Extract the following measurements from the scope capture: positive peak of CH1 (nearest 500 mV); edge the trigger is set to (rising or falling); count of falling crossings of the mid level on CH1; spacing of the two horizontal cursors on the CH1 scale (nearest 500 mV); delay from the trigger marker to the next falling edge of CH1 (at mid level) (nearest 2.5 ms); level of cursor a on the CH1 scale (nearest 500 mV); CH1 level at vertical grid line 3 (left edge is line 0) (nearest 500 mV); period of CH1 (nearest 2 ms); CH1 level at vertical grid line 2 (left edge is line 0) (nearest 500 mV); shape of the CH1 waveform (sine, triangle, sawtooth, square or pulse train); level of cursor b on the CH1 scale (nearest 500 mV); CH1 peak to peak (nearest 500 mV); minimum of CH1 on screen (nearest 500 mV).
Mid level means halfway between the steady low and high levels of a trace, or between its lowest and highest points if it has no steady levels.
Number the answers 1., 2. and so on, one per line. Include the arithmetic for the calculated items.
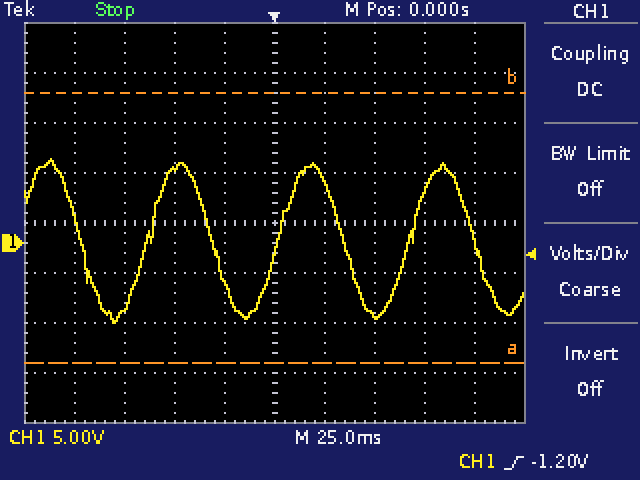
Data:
1. 8.5 V
2. rising
3. 4
4. 27.0 V
5. 35.0 ms
6. -12.0 V
7. 7.5 V
8. 66 ms
9. -6.5 V
10. sine
11. 15.0 V
12. 8.5 V − (-8.0 V) = 16.5 V
13. -8.0 V
